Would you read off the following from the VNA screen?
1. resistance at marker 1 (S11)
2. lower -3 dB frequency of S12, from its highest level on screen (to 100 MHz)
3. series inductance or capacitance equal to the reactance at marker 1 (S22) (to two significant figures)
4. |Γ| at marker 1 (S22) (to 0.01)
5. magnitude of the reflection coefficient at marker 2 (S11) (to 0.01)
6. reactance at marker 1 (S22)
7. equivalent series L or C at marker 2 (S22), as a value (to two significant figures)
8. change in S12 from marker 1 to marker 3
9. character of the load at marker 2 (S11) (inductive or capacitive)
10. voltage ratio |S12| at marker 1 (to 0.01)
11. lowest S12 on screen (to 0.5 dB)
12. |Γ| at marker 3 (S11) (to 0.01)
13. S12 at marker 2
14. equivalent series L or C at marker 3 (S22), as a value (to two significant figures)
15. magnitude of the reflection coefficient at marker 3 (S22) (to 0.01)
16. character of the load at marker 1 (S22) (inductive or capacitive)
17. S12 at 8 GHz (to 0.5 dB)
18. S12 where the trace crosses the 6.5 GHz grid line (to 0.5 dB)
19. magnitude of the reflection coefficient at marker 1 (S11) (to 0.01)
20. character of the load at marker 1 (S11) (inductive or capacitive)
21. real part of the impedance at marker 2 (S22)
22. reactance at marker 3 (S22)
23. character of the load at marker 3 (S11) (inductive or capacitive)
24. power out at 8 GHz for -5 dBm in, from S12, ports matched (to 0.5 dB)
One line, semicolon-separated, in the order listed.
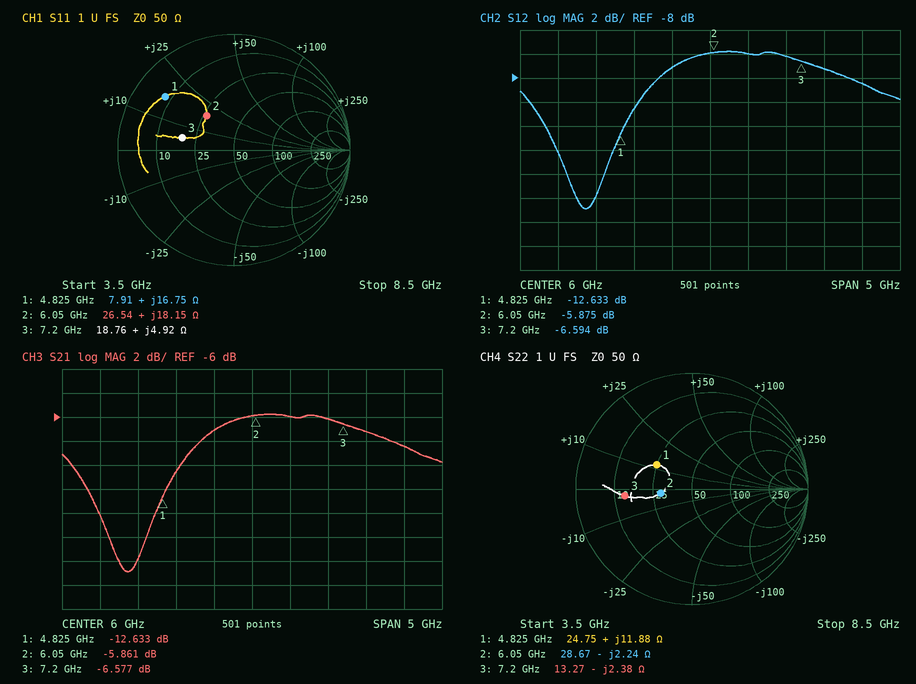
7.91 Ω; 5.2 GHz; 390 pH; 0.37; 0.38; +11.88 Ω; 12 pF; 6.039 dB; inductive; 0.23; -19.0 dB; 0.46; -5.875 dB; 9.3 pF; 0.58; inductive; -8.5 dB; -6.0 dB; 0.75; inductive; 28.67 Ω; -2.38 Ω; inductive; -13.5 dBm
